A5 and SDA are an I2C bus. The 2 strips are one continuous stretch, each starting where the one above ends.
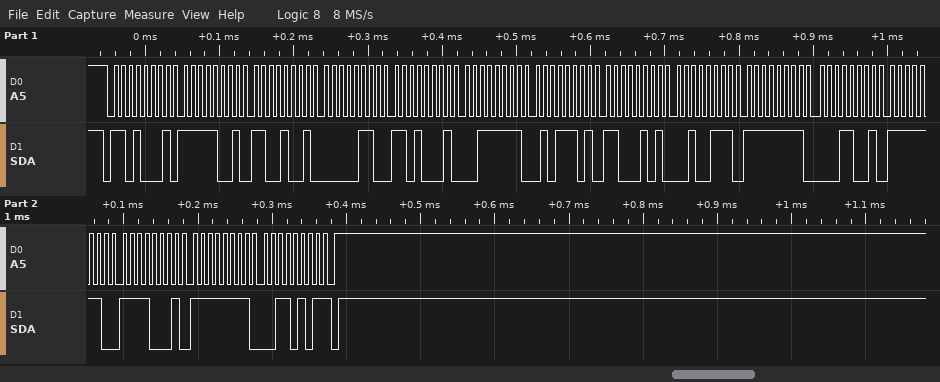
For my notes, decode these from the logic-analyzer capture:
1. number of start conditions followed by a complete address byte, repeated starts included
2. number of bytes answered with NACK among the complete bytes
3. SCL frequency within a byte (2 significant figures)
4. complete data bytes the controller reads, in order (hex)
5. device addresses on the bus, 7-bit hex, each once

1
1
100 kHz
F9 C9 06 D1 3F 5D C5 27 FF 19 FE F1 FF 35
0x68
